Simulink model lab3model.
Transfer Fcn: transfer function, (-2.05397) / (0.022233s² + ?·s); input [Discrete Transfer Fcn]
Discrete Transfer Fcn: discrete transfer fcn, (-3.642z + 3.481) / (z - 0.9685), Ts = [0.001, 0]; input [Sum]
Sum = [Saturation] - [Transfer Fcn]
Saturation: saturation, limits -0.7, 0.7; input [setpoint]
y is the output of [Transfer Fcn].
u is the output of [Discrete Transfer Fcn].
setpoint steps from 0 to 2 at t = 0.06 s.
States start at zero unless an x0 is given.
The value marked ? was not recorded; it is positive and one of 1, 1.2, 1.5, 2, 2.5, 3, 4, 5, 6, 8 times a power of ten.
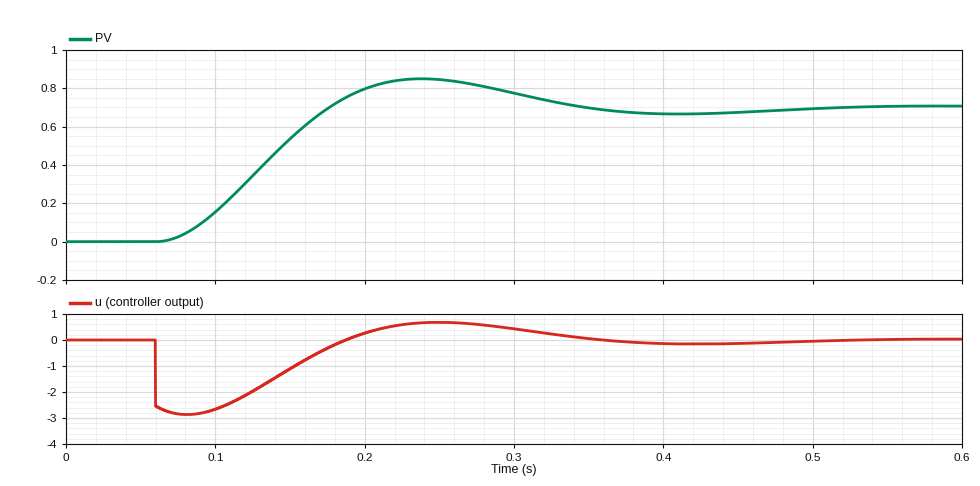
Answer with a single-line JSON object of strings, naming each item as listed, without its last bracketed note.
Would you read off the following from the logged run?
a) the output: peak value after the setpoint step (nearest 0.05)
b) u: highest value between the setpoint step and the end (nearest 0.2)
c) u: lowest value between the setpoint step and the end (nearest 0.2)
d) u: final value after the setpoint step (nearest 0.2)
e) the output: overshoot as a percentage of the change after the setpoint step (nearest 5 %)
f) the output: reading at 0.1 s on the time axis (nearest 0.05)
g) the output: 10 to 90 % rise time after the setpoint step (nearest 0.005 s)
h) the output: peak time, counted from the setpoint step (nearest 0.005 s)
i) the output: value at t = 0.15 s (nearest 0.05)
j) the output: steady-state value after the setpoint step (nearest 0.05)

{"the output: peak value after the setpoint step": "0.85", "u: highest value between the setpoint step and the end": "0.6", "u: lowest value between the setpoint step and the end": "-2.8", "u: final value after the setpoint step": "0.0", "the output: overshoot as a percentage of the change after the setpoint step": "20 %", "the output: reading at 0.1 s on the time axis": "0.15", "the output: 10 to 90 % rise time after the setpoint step": "0.080 s", "the output: peak time, counted from the setpoint step": "0.180 s", "the output: value at t = 0.15 s": "0.55", "the output: steady-state value after the setpoint step": "0.70"}
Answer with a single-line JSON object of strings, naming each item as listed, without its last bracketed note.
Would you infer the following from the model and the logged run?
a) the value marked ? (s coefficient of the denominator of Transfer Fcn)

{"the value marked ?": "0.5"}
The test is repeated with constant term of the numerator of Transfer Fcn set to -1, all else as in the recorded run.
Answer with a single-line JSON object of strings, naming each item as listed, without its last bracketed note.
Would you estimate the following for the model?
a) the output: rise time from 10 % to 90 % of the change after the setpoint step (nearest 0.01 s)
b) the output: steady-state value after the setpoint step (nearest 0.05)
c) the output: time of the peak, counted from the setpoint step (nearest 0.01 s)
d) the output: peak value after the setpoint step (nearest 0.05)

{"the output: rise time from 10 % to 90 % of the change after the setpoint step": "0.14 s", "the output: steady-state value after the setpoint step": "0.70", "the output: time of the peak, counted from the setpoint step": "0.30 s", "the output: peak value after the setpoint step": "0.75"}
